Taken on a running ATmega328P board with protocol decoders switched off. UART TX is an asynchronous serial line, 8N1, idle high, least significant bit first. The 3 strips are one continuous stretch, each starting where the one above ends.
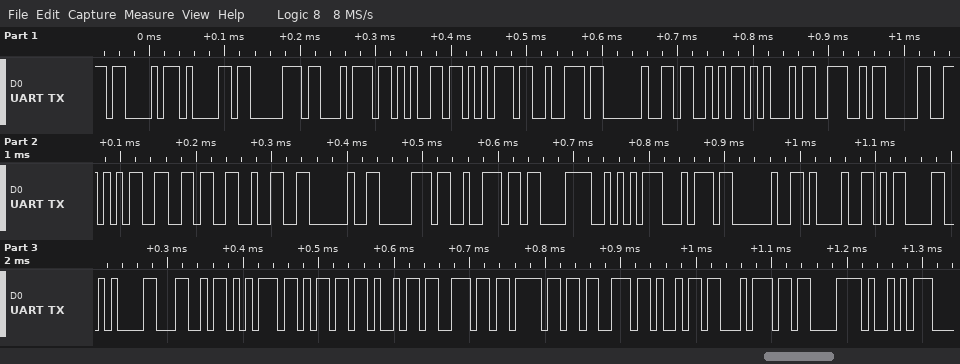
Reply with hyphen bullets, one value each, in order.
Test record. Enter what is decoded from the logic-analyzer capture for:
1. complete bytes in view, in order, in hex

- 43 61 70 74 65 75 72 20 53 45 4E 30 35 36 32 20 70 72 C3 AA 74 20 21 0D 0A 4C 75 6D 69 6E 6F 73 69 74 C3 A9
